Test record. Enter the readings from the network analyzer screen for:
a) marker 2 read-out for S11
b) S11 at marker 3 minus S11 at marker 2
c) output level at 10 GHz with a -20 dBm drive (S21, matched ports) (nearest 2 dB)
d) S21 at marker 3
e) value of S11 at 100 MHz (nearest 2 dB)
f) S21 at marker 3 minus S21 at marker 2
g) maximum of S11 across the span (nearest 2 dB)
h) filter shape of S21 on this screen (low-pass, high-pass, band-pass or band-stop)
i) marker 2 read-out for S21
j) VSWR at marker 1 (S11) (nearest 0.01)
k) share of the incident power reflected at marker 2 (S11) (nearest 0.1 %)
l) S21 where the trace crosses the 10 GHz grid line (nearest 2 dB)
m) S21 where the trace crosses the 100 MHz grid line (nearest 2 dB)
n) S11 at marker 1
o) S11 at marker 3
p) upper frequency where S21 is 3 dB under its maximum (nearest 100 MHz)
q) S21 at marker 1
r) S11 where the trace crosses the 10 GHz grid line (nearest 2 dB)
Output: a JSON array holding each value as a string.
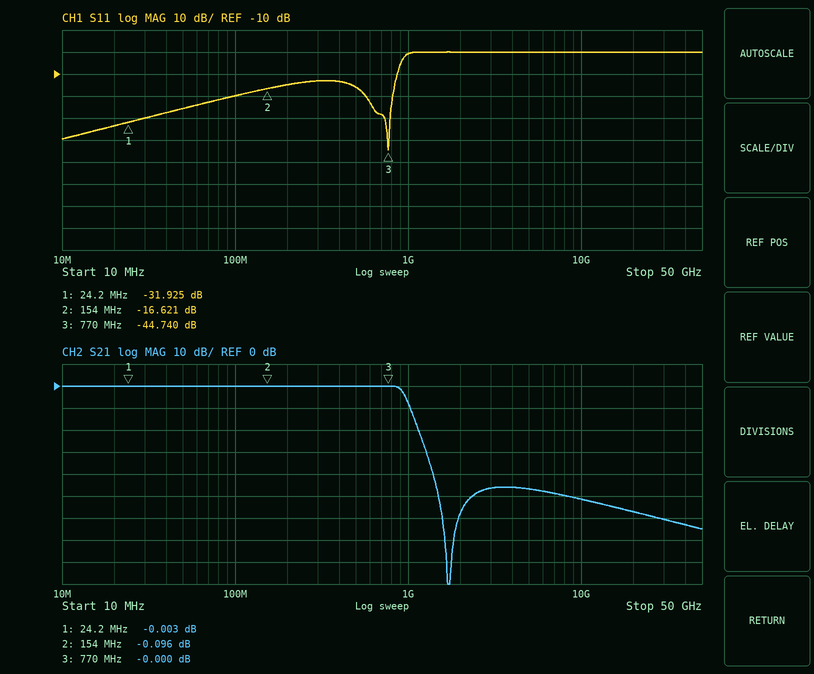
["-16.621 dB", "-28.119 dB", "-72 dBm", "-0.000 dB", "-20 dB", "0.096 dB", "0 dB", "low-pass", "-0.096 dB", "1.05", "2.2 %", "-52 dB", "0 dB", "-31.925 dB", "-44.740 dB", "900 MHz", "-0.003 dB", "0 dB"]
